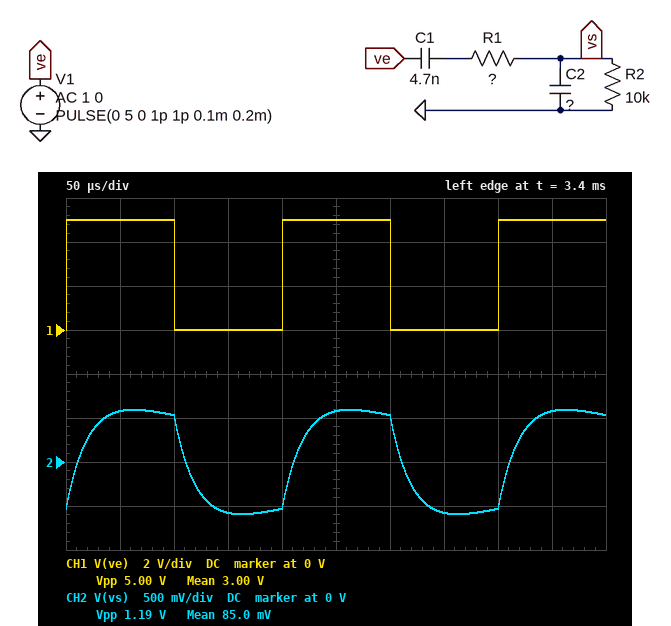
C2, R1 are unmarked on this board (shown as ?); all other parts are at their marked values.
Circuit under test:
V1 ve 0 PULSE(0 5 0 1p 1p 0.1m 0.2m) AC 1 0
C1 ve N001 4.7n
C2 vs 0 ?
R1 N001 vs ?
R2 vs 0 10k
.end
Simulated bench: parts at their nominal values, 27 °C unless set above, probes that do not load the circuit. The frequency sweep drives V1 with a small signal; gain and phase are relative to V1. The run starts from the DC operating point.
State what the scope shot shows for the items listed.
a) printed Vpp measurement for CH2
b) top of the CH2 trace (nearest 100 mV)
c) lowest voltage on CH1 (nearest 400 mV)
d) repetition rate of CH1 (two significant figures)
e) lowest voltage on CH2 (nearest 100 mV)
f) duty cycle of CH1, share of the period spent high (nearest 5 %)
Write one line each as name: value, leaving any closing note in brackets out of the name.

printed Vpp measurement for CH2: 1.19 V
top of the CH2 trace: 600 mV
lowest voltage on CH1: 0 V
repetition rate of CH1: 5.0 kHz
lowest voltage on CH2: -600 mV
duty cycle of CH1, share of the period spent high: 50 %
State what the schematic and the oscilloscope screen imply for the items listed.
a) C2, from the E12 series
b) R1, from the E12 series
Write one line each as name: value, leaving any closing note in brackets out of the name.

C2, from the E12 series: 12 nF
R1, from the E12 series: 6.8 kΩ
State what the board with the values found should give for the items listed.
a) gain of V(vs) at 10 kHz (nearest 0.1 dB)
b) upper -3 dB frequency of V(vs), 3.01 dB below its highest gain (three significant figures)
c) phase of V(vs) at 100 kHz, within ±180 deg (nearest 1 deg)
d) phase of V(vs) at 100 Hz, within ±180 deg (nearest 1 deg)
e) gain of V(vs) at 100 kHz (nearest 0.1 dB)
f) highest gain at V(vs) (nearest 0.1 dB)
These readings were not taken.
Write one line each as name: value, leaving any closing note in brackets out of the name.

gain of V(vs) at 10 kHz: -16.1 dB
upper -3 dB frequency of V(vs), 3.01 dB below its highest gain: 8.99 kHz
phase of V(vs) at 100 kHz, within ±180 deg: -85 deg
phase of V(vs) at 100 Hz, within ±180 deg: 83 deg
gain of V(vs) at 100 kHz: -34.2 dB
highest gain at V(vs): -12.5 dB
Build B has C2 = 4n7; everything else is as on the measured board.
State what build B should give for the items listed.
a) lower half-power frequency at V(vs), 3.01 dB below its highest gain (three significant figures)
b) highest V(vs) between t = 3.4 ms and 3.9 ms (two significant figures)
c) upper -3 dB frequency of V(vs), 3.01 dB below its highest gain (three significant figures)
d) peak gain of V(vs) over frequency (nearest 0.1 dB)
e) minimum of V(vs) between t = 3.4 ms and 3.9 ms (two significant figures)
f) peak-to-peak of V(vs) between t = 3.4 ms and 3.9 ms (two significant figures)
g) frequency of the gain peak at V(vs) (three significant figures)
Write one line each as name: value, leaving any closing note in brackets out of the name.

lower half-power frequency at V(vs), 3.01 dB below its highest gain: 1.16 kHz
highest V(vs) between t = 3.4 ms and 3.9 ms: 1.1 V
upper -3 dB frequency of V(vs), 3.01 dB below its highest gain: 14.5 kHz
peak gain of V(vs) over frequency: -8.6 dB
minimum of V(vs) between t = 3.4 ms and 3.9 ms: -1.1 V
peak-to-peak of V(vs) between t = 3.4 ms and 3.9 ms: 2.1 V
frequency of the gain peak at V(vs): 4.11 kHz
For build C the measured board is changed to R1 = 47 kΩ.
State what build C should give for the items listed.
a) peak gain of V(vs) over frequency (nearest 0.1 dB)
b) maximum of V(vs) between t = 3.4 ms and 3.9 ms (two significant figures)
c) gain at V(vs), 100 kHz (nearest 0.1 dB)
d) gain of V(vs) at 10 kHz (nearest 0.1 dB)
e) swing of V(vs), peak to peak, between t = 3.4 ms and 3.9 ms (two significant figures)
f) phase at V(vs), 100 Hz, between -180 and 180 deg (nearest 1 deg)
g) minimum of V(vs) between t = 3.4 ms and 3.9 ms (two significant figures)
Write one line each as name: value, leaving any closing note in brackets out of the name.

peak gain of V(vs) over frequency: -18.3 dB
maximum of V(vs) between t = 3.4 ms and 3.9 ms: 190 mV
gain at V(vs), 100 kHz: -51.0 dB
gain of V(vs) at 10 kHz: -31.1 dB
swing of V(vs), peak to peak, between t = 3.4 ms and 3.9 ms: 390 mV
phase at V(vs), 100 Hz, between -180 and 180 deg: 76 deg
minimum of V(vs) between t = 3.4 ms and 3.9 ms: -190 mV
